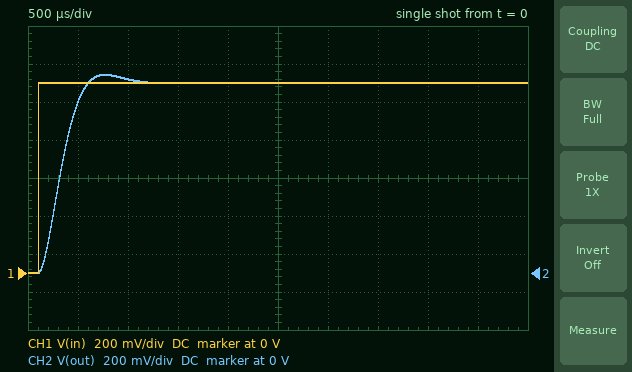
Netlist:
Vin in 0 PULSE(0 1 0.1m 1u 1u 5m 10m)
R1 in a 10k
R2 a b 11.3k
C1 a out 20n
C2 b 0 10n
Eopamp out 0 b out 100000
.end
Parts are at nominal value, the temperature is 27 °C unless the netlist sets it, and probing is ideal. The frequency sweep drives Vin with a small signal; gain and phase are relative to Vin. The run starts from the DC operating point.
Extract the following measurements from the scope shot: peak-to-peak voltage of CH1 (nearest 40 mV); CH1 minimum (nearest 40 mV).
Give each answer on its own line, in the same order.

1.00 V
0 V
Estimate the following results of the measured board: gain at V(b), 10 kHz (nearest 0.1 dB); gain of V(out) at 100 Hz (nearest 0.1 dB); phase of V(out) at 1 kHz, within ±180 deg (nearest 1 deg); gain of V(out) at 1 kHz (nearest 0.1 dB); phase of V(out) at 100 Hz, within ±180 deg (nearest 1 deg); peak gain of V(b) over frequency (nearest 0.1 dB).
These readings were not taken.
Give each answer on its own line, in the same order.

-39.0 dB
0 dB
-85 deg
-2.6 dB
-8 deg
0 dB
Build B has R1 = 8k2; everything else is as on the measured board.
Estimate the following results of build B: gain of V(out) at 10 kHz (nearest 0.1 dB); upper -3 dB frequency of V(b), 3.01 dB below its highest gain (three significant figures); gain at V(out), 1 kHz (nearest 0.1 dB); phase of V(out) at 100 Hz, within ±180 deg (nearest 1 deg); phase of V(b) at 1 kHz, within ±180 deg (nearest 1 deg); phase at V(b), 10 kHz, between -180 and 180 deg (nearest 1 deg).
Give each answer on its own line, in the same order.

-37.3 dB
1.15 kHz
-2.0 dB
-7 deg
-78 deg
-170 deg
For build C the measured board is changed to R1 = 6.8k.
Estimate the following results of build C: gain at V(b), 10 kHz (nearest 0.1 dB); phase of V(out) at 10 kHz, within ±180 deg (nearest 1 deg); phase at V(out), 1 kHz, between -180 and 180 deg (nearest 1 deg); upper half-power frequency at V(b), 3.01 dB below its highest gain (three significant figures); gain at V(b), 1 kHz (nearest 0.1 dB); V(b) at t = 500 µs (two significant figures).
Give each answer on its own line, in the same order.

-35.7 dB
-169 deg
-71 deg
1.24 kHz
-1.6 dB
970 mV
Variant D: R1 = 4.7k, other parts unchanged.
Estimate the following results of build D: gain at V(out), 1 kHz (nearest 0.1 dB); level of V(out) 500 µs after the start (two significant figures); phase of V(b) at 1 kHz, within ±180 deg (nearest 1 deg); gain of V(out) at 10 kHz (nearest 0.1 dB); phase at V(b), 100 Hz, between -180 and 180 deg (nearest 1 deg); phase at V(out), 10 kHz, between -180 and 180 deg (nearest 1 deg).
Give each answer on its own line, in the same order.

-1.3 dB
1.0 V
-60 deg
-32.5 dB
-6 deg
-166 deg
